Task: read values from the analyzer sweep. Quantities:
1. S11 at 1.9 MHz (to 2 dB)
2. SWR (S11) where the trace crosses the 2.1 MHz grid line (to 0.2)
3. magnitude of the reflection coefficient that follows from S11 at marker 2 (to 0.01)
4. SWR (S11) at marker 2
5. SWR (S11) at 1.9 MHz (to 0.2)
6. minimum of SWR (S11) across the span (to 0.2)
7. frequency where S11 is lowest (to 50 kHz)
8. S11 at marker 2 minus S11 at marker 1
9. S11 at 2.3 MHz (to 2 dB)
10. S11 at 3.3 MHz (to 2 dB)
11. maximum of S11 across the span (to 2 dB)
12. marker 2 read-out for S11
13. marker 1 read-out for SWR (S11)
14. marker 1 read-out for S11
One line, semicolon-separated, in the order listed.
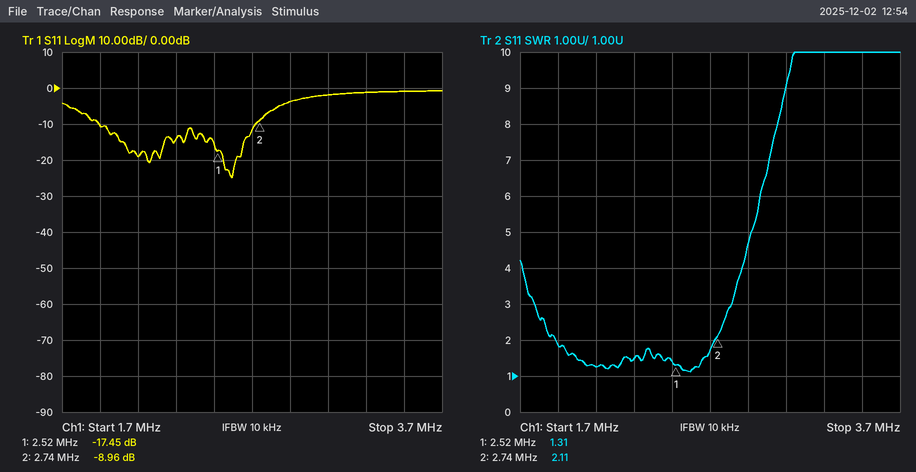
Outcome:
-10 dB; 1.2; 0.36; 2.11; 1.8; 1.2; 2.60 MHz; 8.49 dB; -14 dB; -2 dB; 0 dB; -8.96 dB; 1.31; -17.45 dB
